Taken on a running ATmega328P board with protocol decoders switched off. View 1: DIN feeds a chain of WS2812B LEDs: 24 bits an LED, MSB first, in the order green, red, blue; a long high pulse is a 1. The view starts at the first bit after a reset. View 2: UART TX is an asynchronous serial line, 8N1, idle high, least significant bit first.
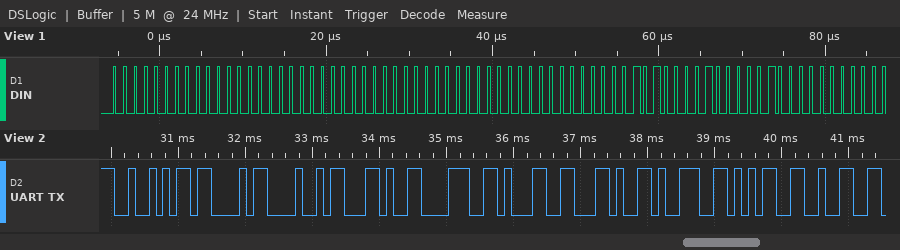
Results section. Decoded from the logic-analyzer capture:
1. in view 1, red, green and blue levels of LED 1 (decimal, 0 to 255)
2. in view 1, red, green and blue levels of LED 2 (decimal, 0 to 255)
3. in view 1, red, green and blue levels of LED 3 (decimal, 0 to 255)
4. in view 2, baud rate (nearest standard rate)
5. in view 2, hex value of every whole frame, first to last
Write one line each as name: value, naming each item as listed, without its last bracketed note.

in view 1, red, green and blue levels of LED 1: 0, 0, 0
in view 1, red, green and blue levels of LED 2: 0, 0, 0
in view 1, red, green and blue levels of LED 3: 65, 40, 0
in view 2, baud rate: 9600 baud
in view 2, hex value of every whole frame, first to last: 0x52 0x43 0x48 0x2C 0x38 0x31 0x2C 0x39 0x35 0x32
